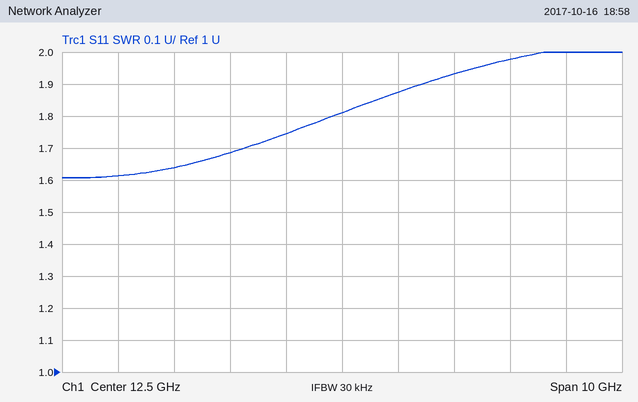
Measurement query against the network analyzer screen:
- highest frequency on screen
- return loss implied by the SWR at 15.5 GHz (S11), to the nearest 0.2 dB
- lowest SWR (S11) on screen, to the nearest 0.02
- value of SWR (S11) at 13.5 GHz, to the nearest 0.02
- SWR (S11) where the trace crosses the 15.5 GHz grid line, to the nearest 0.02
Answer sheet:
17.5 GHz
9.6 dB
1.60
1.88
1.98
